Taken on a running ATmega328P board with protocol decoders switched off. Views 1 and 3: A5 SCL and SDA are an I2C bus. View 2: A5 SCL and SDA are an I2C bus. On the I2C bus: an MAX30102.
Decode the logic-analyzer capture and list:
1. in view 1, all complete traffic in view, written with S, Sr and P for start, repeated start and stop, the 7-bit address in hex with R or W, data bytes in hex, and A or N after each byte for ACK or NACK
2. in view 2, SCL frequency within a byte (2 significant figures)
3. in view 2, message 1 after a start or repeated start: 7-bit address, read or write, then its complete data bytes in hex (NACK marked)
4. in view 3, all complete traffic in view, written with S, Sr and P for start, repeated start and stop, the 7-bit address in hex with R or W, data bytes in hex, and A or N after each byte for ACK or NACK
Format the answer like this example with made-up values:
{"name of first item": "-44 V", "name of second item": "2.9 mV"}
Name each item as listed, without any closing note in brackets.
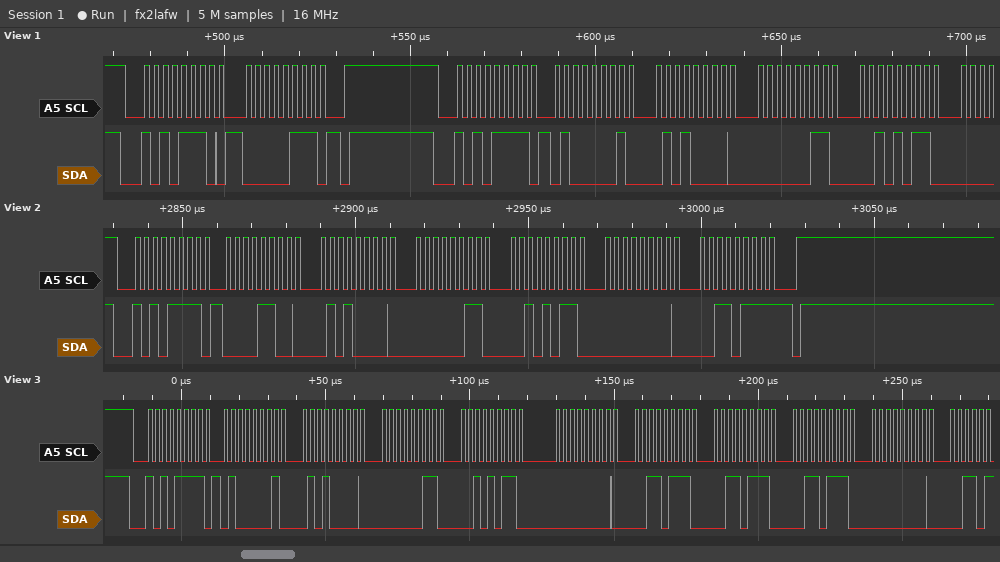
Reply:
{"in view 1, all complete traffic in view, written with S, Sr and P for start, repeated start and stop, the 7-bit address in hex with R or W, data bytes in hex, and A or N after each byte for ACK or NACK": "S 57W A 07 A P S 57R A 41 A 50 A 03 A 2B A", "in view 2, SCL frequency within a byte": "400 kHz", "in view 2, message 1 after a start or repeated start: 7-bit address, read or write, then its complete data bytes in hex": "0x57 read: 0C 50 03 2B 00 37 NACK", "in view 3, all complete traffic in view, written with S, Sr and P for start, repeated start and stop, the 7-bit address in hex with R or W, data bytes in hex, and A or N after each byte for ACK or NACK": "S 57R A 41 A 50 A 03 A 2B A 00 A 37 A 37 A 37 A 00 A"}
